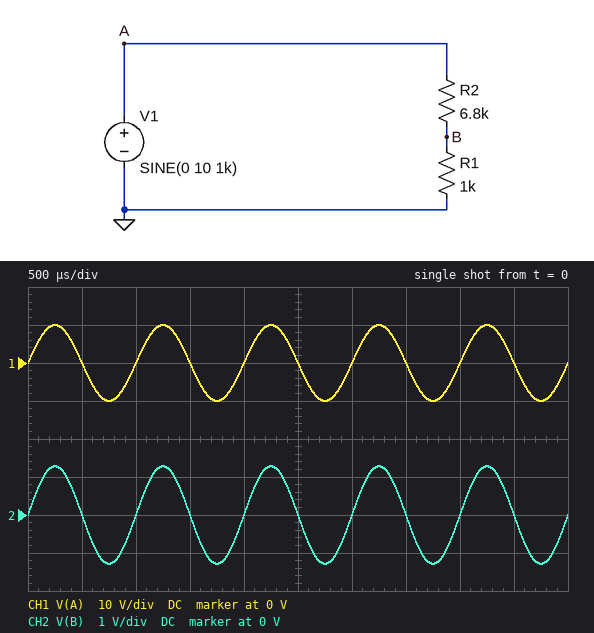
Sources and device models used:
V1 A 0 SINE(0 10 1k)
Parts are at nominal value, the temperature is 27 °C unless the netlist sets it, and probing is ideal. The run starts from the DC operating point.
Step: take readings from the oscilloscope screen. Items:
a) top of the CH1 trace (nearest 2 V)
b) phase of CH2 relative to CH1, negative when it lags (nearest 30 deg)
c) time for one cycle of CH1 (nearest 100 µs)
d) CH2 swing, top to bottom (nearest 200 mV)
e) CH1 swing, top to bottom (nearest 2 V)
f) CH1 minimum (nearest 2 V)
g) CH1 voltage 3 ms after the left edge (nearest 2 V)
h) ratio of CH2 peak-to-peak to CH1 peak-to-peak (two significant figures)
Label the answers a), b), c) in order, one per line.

a) 10 V
b) 0 deg
c) 1.0 ms
d) 2.6 V
e) 20 V
f) -10 V
g) 0 V
h) 0.13
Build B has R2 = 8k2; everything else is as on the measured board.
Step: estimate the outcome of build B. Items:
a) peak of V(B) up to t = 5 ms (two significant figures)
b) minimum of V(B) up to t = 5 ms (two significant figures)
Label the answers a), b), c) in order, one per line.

a) 1.1 V
b) -1.1 V
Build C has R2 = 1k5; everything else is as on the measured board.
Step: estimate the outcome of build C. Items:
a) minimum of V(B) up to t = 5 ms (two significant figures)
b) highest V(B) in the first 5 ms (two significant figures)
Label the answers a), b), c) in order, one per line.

a) -4.0 V
b) 4.0 V
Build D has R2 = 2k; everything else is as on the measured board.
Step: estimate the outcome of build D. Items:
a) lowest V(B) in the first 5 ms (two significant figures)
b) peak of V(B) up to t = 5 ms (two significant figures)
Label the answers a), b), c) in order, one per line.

a) -3.3 V
b) 3.3 V
